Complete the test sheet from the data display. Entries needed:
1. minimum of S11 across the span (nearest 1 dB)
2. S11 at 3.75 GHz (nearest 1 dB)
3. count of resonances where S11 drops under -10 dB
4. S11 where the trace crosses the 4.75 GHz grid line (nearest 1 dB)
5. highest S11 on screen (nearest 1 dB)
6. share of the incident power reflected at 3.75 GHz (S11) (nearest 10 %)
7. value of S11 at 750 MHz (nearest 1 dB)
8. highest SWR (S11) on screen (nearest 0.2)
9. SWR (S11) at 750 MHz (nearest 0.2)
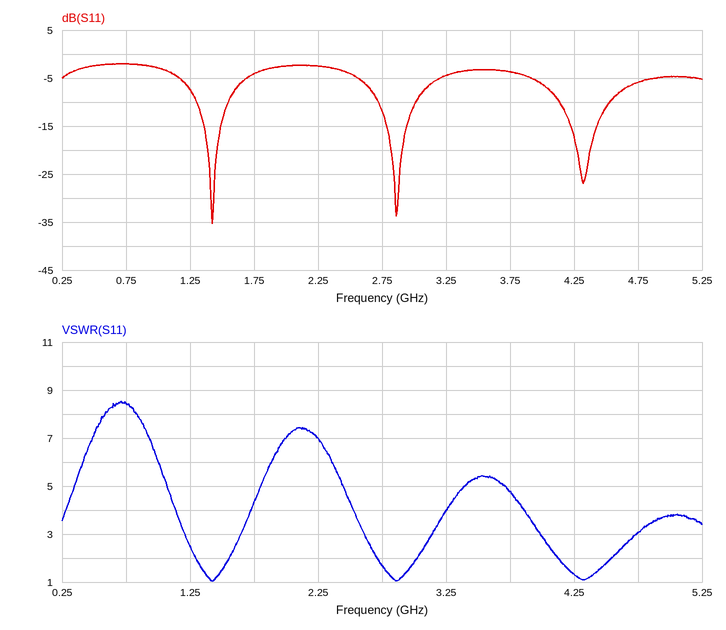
-35 dB
-4 dB
3
-6 dB
-2 dB
40 %
-2 dB
8.6
8.4
